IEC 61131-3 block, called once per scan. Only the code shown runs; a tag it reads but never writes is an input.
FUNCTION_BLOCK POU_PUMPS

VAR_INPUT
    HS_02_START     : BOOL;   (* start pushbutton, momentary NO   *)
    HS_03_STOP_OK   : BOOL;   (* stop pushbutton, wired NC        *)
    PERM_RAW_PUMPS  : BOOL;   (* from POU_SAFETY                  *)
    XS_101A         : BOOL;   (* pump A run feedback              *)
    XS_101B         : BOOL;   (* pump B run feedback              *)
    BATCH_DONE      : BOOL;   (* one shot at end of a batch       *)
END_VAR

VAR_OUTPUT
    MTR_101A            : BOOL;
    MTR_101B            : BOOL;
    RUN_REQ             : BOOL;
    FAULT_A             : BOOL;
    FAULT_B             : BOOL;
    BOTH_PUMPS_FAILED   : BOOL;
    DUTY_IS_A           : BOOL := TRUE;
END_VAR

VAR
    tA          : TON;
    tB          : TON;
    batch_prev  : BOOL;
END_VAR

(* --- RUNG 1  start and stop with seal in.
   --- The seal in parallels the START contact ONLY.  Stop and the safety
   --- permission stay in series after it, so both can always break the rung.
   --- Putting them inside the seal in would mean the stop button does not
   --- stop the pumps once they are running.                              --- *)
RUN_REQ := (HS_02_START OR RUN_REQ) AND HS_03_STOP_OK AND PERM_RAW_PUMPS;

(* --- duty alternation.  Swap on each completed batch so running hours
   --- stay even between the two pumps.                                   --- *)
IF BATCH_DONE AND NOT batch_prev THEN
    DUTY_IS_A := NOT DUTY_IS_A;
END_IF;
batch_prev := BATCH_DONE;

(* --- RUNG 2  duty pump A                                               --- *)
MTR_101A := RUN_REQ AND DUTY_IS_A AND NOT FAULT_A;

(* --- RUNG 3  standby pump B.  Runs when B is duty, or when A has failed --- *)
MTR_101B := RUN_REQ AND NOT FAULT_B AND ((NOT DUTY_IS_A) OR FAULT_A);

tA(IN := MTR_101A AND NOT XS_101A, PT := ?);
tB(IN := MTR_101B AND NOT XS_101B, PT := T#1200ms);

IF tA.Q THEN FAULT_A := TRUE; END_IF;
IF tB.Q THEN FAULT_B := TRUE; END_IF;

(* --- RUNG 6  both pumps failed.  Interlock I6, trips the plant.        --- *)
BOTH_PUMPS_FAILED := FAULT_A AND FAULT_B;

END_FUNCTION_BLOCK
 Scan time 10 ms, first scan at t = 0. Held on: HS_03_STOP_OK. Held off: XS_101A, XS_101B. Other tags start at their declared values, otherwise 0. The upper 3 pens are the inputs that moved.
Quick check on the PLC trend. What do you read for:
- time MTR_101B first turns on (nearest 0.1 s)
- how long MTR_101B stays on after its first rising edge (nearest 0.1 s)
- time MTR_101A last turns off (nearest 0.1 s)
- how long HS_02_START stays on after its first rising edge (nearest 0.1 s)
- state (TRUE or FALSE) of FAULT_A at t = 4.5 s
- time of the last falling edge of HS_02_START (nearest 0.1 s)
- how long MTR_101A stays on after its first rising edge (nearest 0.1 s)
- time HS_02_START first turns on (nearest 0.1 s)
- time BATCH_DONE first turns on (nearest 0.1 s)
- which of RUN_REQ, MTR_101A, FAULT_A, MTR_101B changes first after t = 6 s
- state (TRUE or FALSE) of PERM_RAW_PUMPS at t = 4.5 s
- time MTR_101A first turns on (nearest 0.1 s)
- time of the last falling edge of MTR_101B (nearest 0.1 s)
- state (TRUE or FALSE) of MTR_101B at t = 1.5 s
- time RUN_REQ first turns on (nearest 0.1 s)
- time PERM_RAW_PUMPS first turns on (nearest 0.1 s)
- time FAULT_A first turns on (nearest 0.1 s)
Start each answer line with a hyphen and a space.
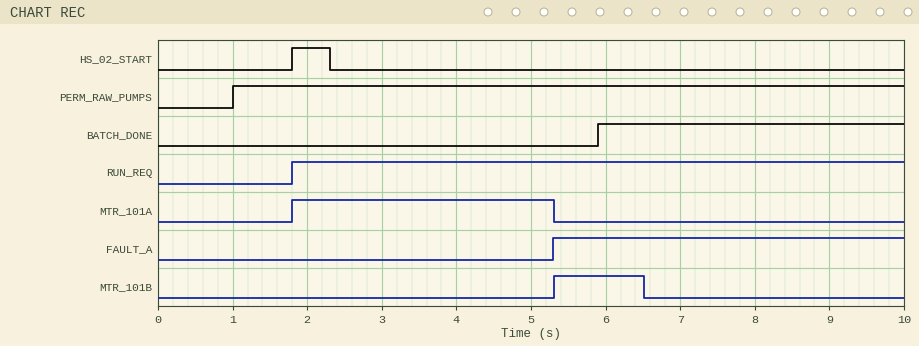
- 5.3 s
- 1.2 s
- 5.3 s
- 0.5 s
- FALSE
- 2.3 s
- 3.5 s
- 1.8 s
- 5.9 s
- MTR_101B
- TRUE
- 1.8 s
- 6.5 s
- FALSE
- 1.8 s
- 1.0 s
- 5.3 s
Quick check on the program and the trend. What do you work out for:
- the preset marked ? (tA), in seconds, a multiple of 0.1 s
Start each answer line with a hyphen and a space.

- 3.5 s
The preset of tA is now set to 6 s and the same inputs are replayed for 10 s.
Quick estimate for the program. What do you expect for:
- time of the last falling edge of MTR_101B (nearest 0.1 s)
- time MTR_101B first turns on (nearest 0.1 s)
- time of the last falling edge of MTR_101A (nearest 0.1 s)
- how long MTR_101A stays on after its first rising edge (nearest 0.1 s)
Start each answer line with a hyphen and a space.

- 7.1 s
- 5.9 s
- 5.9 s
- 4.1 s
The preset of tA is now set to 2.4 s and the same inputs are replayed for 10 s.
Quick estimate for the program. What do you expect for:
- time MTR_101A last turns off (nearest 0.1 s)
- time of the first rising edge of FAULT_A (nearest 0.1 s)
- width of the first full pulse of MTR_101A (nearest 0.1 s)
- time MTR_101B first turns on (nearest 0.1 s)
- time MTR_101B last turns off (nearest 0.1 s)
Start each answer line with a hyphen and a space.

- 4.2 s
- 4.2 s
- 2.4 s
- 4.2 s
- 5.4 s
